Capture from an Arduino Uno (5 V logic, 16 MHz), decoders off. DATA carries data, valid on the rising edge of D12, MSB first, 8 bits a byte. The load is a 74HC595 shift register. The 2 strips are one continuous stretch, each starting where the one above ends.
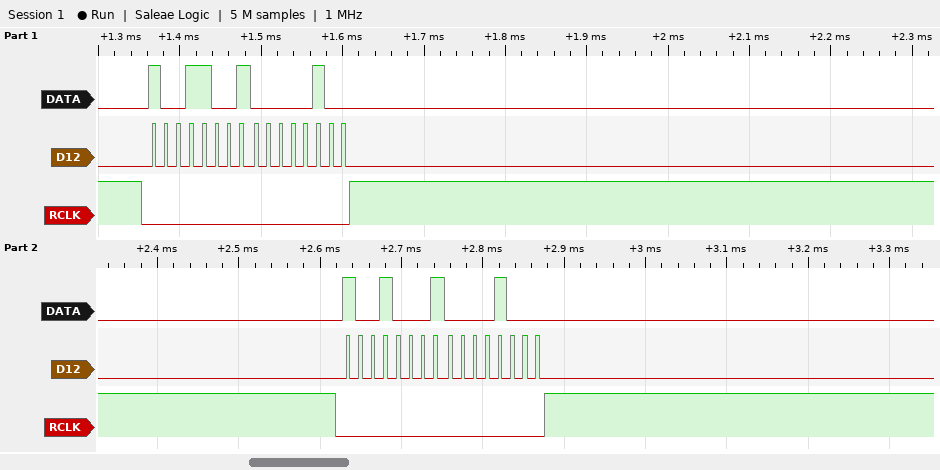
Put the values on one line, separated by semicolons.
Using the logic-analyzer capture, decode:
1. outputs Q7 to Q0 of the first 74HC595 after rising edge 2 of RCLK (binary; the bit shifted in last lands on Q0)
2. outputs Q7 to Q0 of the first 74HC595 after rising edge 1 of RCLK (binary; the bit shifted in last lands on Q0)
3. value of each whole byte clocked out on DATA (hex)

00001000; 00000100; 0x99 0x04 0x91 0x08
